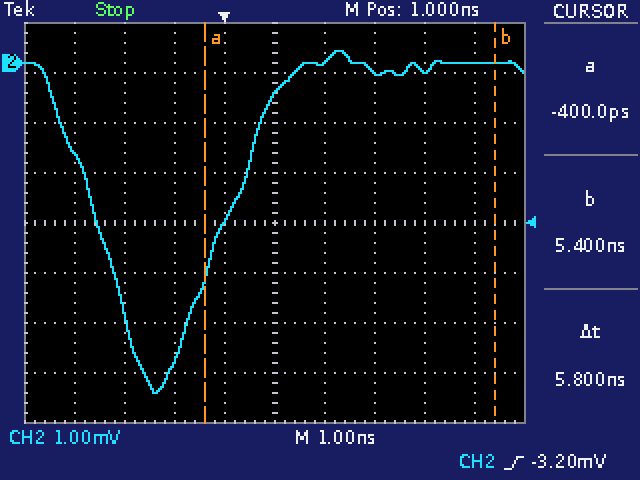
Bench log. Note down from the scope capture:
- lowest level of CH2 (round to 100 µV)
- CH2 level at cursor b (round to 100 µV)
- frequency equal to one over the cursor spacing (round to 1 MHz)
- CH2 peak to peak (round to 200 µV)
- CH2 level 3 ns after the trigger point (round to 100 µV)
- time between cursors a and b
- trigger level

-6.6 mV
0.0 mV
172 MHz
6.8 mV
-200 µV
5.8 ns
-3.20 mV
